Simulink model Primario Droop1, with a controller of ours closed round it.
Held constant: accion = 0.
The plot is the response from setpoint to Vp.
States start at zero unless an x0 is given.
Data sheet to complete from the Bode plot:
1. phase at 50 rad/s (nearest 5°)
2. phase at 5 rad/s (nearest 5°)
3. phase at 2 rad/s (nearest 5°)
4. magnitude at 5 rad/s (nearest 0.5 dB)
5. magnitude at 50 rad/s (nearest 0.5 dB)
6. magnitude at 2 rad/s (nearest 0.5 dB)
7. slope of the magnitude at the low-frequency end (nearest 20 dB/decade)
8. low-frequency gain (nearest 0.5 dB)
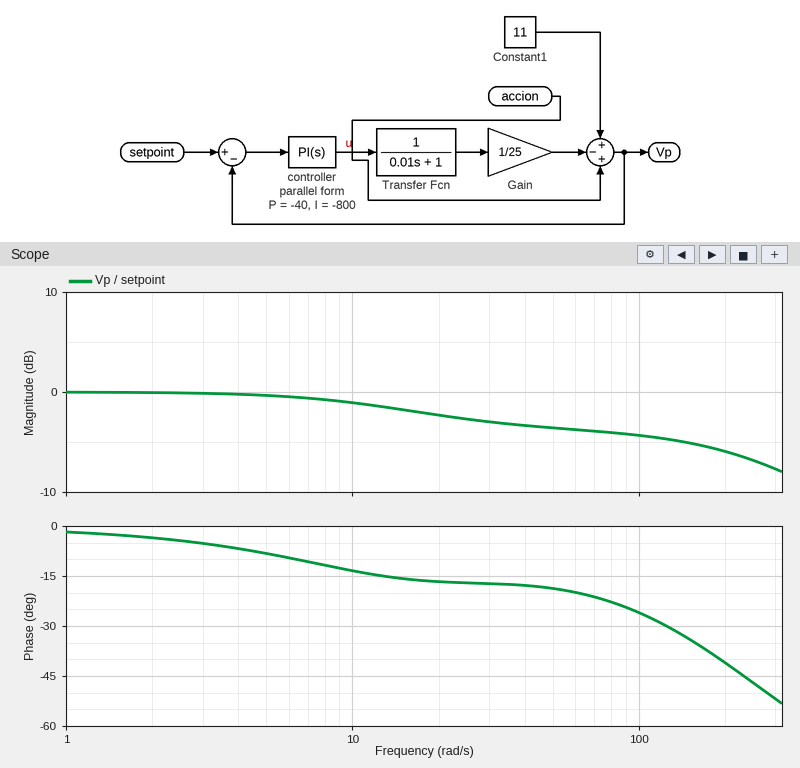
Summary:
-20°
-10°
-5°
-0.5 dB
-3.5 dB
0.0 dB
0 dB/decade
0.0 dB
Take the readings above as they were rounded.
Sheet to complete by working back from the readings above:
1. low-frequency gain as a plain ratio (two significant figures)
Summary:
1.0
